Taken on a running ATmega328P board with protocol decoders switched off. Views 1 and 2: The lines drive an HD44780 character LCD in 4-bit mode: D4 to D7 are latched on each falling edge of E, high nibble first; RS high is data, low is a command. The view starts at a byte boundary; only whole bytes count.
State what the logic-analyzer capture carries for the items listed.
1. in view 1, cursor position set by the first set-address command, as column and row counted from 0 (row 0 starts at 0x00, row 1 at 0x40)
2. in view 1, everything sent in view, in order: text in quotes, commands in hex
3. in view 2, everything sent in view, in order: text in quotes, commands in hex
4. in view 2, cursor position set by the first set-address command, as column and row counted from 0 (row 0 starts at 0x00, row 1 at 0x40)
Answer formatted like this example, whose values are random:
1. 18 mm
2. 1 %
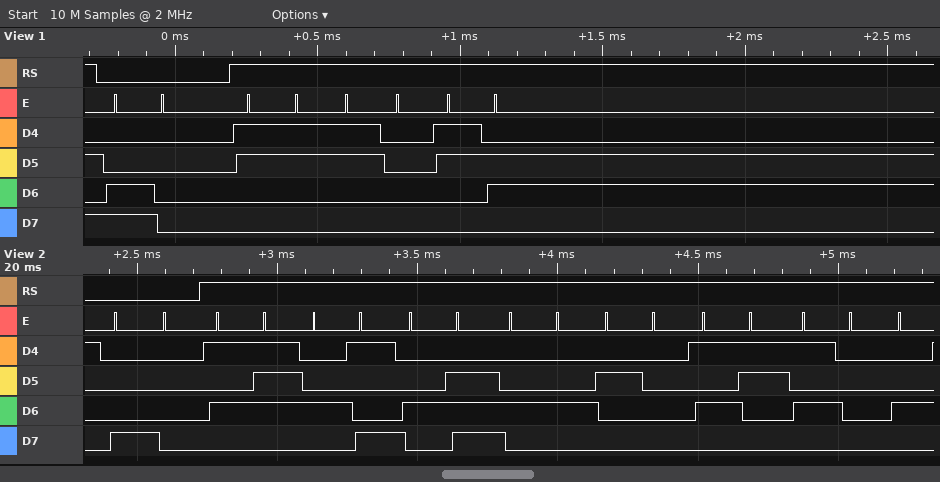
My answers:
1. column 0, row 1
2. 0xC0 "306"
3. 0x80 "WIND SP"
4. column 0, row 0
